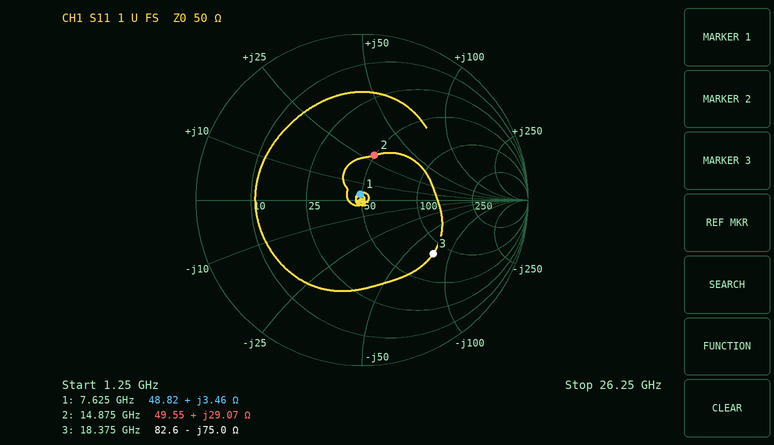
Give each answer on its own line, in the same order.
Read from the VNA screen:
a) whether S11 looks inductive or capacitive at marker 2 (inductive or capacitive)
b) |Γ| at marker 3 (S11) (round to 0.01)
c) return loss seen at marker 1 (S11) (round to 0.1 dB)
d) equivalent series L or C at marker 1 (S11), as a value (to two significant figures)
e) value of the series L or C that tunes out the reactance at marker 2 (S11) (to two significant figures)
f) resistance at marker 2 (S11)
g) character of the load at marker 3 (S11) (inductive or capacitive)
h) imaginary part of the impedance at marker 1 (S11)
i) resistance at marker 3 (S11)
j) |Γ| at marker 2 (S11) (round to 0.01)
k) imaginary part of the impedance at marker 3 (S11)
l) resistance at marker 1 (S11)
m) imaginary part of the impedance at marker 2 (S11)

inductive
0.54
28.6 dB
72 pH
370 fF
49.55 Ω
capacitive
+3.46 Ω
82.6 Ω
0.28
-75.0 Ω
48.82 Ω
+29.07 Ω
